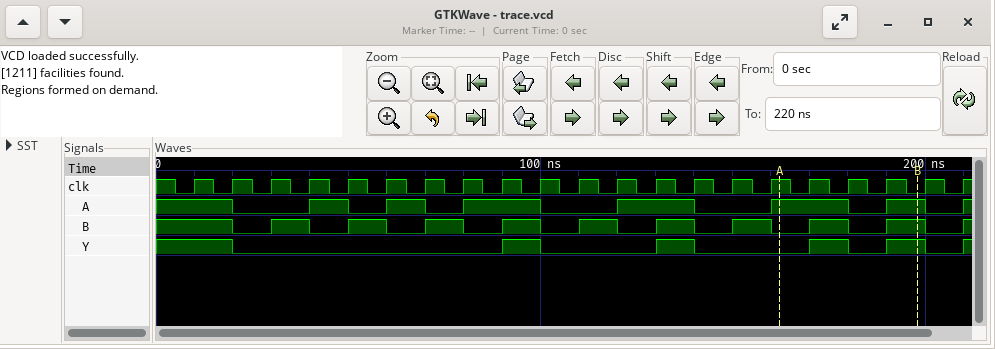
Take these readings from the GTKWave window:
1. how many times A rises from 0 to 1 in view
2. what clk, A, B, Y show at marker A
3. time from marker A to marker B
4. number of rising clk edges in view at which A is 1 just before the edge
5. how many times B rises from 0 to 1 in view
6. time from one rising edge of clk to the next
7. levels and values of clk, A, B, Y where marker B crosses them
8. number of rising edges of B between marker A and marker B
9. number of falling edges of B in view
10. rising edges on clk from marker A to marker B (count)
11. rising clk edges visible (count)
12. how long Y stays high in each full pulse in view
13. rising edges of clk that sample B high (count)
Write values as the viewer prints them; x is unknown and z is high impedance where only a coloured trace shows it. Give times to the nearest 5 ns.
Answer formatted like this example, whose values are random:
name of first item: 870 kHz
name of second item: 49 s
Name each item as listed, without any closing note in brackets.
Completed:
how many times A rises from 0 to 1 in view: 7
what clk, A, B, Y show at marker A: clk=1, A=1, B=0, Y=0
time from marker A to marker B: 35 ns
number of rising clk edges in view at which A is 1 just before the edge: 11
how many times B rises from 0 to 1 in view: 10
time from one rising edge of clk to the next: 10 ns
levels and values of clk, A, B, Y where marker B crosses them: clk=0, A=1, B=1, Y=1
number of rising edges of B between marker A and marker B: 2
number of falling edges of B in view: 10
rising edges on clk from marker A to marker B: 3
rising clk edges visible: 21
how long Y stays high in each full pulse in view: 10 ns, 10 ns, 10 ns, 10 ns
rising edges of clk that sample B high: 11
